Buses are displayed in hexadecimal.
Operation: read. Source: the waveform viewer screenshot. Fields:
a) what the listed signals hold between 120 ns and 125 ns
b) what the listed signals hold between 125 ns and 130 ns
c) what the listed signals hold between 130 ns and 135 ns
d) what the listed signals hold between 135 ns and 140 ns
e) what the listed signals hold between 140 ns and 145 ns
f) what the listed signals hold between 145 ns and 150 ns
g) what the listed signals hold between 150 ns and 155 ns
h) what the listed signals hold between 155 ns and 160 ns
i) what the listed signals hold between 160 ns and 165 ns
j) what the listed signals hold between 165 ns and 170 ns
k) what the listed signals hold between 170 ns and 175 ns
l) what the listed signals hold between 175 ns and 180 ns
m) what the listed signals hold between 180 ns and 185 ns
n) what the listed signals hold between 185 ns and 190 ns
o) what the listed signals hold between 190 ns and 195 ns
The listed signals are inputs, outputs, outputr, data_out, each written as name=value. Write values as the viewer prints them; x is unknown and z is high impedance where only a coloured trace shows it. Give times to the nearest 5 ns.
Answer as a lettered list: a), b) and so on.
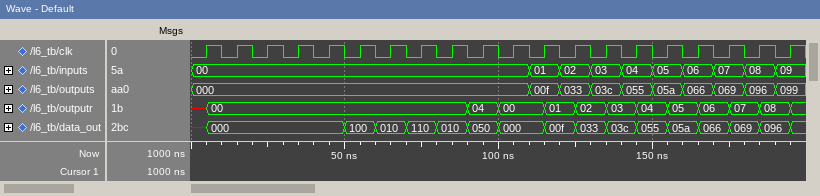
a) inputs=02, outputs=033, outputr=01, data_out=00f
b) inputs=02, outputs=033, outputr=02, data_out=033
c) inputs=03, outputs=03c, outputr=02, data_out=033
d) inputs=03, outputs=03c, outputr=03, data_out=03c
e) inputs=04, outputs=055, outputr=03, data_out=03c
f) inputs=04, outputs=055, outputr=04, data_out=055
g) inputs=05, outputs=05a, outputr=04, data_out=055
h) inputs=05, outputs=05a, outputr=05, data_out=05a
i) inputs=06, outputs=066, outputr=05, data_out=05a
j) inputs=06, outputs=066, outputr=06, data_out=066
k) inputs=07, outputs=069, outputr=06, data_out=066
l) inputs=07, outputs=069, outputr=07, data_out=069
m) inputs=08, outputs=096, outputr=07, data_out=069
n) inputs=08, outputs=096, outputr=08, data_out=096
o) inputs=09, outputs=099, outputr=08, data_out=096
